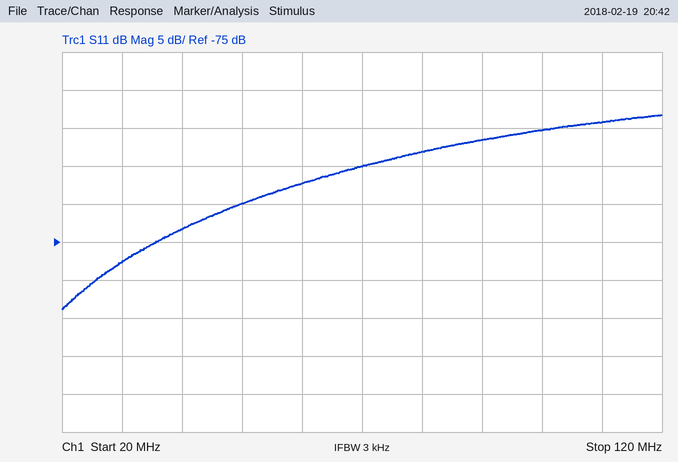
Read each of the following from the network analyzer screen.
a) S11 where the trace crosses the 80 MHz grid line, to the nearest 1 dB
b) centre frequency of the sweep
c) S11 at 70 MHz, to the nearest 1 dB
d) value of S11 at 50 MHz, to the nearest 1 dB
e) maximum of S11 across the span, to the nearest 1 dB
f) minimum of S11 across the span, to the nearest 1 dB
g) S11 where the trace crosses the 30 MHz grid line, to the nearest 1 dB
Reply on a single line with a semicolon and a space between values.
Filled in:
-63 dB; 70 MHz; -65 dB; -70 dB; -58 dB; -84 dB; -78 dB
